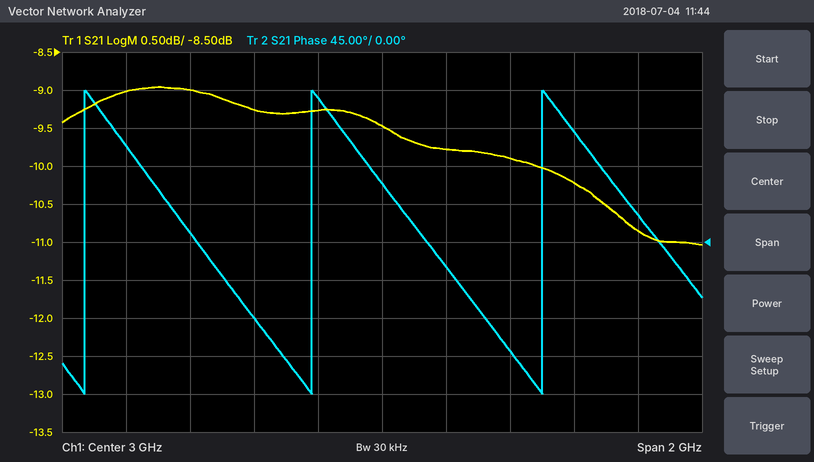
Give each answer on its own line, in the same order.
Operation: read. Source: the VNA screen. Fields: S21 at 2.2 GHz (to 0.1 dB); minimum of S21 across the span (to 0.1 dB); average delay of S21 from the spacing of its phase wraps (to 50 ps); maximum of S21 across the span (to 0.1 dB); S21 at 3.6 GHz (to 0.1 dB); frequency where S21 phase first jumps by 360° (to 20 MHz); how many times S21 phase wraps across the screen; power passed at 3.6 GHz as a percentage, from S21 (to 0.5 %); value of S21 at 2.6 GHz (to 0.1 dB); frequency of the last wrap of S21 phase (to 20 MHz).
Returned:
-9.0 dB
-11.0 dB
1.40 ns
-9.0 dB
-10.2 dB
2.08 GHz
3
9.5 %
-9.3 dB
3.50 GHz
